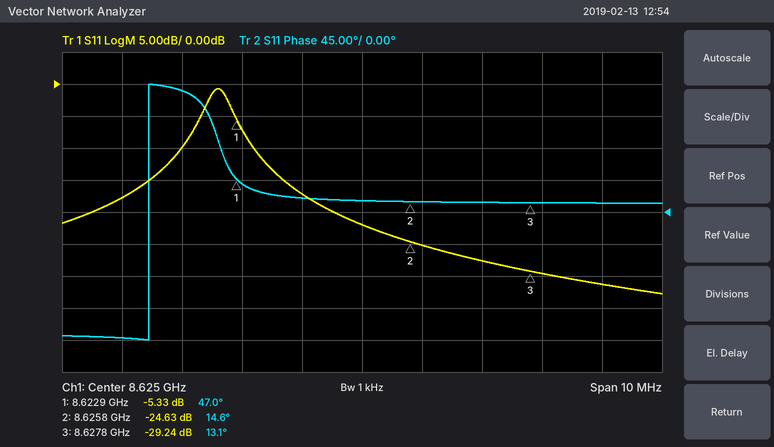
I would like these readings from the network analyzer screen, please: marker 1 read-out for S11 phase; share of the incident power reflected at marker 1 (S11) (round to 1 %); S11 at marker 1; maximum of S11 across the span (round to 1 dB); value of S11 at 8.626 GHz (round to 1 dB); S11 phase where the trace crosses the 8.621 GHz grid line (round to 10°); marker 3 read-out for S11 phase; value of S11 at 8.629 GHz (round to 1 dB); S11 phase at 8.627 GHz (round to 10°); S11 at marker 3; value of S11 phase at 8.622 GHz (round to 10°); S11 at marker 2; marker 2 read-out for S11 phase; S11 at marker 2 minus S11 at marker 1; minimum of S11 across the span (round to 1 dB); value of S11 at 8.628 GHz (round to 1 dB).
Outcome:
47.0°
29 %
-5.33 dB
-1 dB
-25 dB
-180°
13.1°
-31 dB
10°
-29.24 dB
170°
-24.63 dB
14.6°
-19.30 dB
-33 dB
-30 dB
